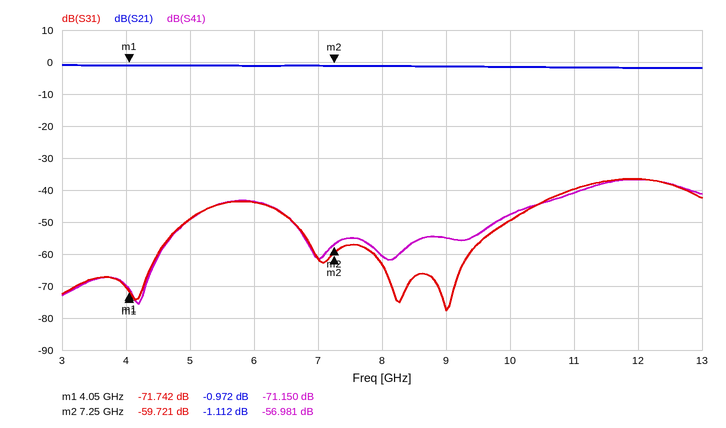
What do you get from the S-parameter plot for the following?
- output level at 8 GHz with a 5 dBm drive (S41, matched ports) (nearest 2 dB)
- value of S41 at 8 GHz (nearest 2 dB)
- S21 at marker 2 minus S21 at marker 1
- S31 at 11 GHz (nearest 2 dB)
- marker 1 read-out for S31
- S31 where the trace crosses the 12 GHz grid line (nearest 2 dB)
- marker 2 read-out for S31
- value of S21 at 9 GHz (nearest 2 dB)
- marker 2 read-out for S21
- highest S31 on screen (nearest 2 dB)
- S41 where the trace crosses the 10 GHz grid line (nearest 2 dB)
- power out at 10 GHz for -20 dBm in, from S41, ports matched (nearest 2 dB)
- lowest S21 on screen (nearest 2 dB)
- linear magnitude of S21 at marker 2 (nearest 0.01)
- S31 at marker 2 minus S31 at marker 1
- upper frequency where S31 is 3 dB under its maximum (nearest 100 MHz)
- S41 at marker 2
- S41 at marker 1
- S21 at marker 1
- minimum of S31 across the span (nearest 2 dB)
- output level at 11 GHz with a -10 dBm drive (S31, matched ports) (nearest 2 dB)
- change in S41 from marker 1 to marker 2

-56 dBm
-60 dB
-0.140 dB
-40 dB
-71.742 dB
-36 dB
-59.721 dB
-2 dB
-1.112 dB
-36 dB
-48 dB
-68 dBm
-2 dB
0.88
12.021 dB
12.7 GHz
-56.981 dB
-71.150 dB
-0.972 dB
-78 dB
-50 dBm
14.169 dB
